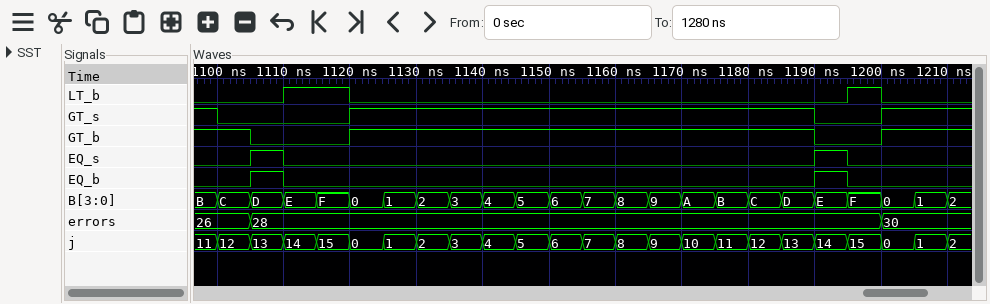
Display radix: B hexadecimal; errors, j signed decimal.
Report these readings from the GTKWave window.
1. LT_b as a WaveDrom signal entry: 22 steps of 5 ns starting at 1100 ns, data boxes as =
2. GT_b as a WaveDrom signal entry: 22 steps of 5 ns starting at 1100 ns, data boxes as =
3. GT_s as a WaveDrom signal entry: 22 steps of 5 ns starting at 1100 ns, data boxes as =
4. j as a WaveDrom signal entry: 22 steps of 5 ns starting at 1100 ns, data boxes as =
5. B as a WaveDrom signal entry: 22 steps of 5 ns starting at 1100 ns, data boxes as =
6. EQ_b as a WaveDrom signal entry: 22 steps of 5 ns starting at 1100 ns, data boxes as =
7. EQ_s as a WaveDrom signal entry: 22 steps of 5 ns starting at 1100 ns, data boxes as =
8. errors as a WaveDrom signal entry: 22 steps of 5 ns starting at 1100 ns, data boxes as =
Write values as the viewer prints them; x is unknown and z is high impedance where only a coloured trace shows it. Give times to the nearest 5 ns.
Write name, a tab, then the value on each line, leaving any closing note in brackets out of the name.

LT_b as a WaveDrom signal entry: 22 steps of 5 ns starting at 1100 ns, data boxes as =	{name: 'LT_b', wave: '0.1.0..............10.'}
GT_b as a WaveDrom signal entry: 22 steps of 5 ns starting at 1100 ns, data boxes as =	{name: 'GT_b', wave: '10..1.............0.1.'}
GT_s as a WaveDrom signal entry: 22 steps of 5 ns starting at 1100 ns, data boxes as =	{name: 'GT_s', wave: '0...1.............0.1.'}
j as a WaveDrom signal entry: 22 steps of 5 ns starting at 1100 ns, data boxes as =	{name: 'j', wave: '======================', data: '12 13 14 15 0 1 2 3 4 5 6 7 8 9 10 11 12 13 14 15 0 1'}
B as a WaveDrom signal entry: 22 steps of 5 ns starting at 1100 ns, data boxes as =	{name: 'B', wave: '======================', data: 'C D E F 0 1 2 3 4 5 6 7 8 9 A B C D E F 0 1'}
EQ_b as a WaveDrom signal entry: 22 steps of 5 ns starting at 1100 ns, data boxes as =	{name: 'EQ_b', wave: '010...............10..'}
EQ_s as a WaveDrom signal entry: 22 steps of 5 ns starting at 1100 ns, data boxes as =	{name: 'EQ_s', wave: '010...............10..'}
errors as a WaveDrom signal entry: 22 steps of 5 ns starting at 1100 ns, data boxes as =	{name: 'errors', wave: '==..................=.', data: '26 28 30'}
